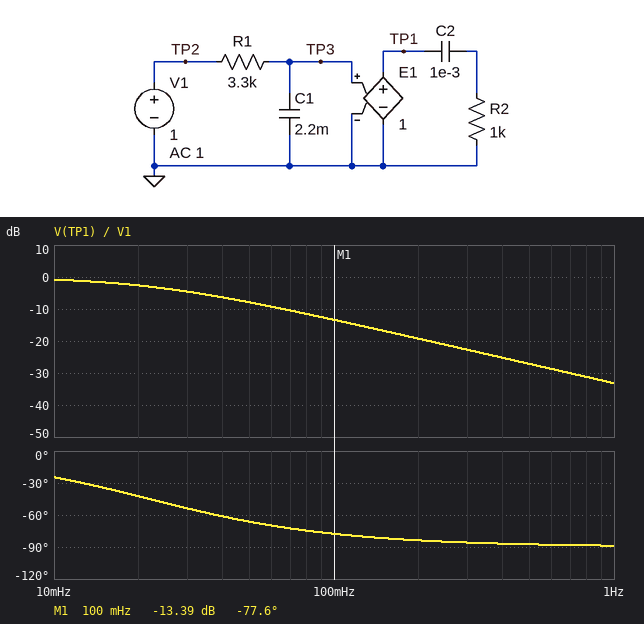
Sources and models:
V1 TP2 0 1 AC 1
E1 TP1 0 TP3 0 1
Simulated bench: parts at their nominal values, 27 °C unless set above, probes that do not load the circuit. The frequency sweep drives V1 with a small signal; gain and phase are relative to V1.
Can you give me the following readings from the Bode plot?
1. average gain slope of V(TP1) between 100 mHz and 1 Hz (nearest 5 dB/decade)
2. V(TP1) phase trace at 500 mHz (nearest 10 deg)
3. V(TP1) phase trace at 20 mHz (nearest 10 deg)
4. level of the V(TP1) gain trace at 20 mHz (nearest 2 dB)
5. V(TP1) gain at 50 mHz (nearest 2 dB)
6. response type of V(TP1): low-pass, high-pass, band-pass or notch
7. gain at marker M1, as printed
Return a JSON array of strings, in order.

["-20 dB/decade", "-90 deg", "-40 deg", "-2 dB", "-8 dB", "low-pass", "-13.39 dB"]
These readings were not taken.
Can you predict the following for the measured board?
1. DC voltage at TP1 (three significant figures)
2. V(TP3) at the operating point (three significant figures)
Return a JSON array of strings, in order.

["1.00 V", "1.00 V"]
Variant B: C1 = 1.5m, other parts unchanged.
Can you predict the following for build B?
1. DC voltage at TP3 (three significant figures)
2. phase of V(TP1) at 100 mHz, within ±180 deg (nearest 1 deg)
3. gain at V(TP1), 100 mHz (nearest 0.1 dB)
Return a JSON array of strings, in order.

["1.00 V", "-72 deg", "-10.3 dB"]
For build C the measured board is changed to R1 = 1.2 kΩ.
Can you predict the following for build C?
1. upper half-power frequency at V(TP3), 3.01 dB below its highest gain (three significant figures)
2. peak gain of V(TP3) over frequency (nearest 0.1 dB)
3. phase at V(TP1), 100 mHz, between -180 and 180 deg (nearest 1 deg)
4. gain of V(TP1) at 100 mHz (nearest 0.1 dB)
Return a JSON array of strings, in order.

["60.3 mHz", "0 dB", "-59 deg", "-5.7 dB"]
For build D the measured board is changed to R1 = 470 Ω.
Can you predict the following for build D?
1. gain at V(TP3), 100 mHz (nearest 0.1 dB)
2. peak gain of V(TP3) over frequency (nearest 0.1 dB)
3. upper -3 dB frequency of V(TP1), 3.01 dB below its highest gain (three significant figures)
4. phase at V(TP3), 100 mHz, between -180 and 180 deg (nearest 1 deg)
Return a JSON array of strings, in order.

["-1.5 dB", "0 dB", "154 mHz", "-33 deg"]
